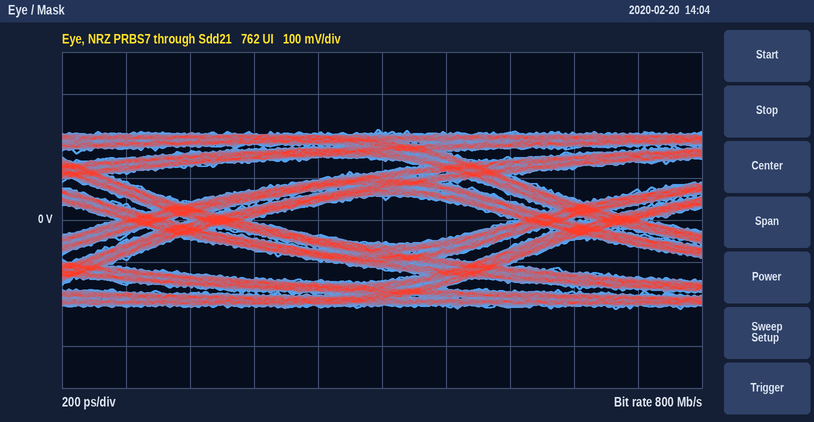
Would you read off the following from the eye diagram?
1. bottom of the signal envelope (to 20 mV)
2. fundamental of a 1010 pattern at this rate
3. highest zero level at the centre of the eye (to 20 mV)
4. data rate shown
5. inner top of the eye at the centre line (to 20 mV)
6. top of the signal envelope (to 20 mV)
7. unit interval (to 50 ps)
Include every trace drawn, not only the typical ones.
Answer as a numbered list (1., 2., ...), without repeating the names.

1. -220 mV
2. 400 MHz
3. -60 mV
4. 800 Mb/s
5. 60 mV
6. 220 mV
7. 1.25 ns
